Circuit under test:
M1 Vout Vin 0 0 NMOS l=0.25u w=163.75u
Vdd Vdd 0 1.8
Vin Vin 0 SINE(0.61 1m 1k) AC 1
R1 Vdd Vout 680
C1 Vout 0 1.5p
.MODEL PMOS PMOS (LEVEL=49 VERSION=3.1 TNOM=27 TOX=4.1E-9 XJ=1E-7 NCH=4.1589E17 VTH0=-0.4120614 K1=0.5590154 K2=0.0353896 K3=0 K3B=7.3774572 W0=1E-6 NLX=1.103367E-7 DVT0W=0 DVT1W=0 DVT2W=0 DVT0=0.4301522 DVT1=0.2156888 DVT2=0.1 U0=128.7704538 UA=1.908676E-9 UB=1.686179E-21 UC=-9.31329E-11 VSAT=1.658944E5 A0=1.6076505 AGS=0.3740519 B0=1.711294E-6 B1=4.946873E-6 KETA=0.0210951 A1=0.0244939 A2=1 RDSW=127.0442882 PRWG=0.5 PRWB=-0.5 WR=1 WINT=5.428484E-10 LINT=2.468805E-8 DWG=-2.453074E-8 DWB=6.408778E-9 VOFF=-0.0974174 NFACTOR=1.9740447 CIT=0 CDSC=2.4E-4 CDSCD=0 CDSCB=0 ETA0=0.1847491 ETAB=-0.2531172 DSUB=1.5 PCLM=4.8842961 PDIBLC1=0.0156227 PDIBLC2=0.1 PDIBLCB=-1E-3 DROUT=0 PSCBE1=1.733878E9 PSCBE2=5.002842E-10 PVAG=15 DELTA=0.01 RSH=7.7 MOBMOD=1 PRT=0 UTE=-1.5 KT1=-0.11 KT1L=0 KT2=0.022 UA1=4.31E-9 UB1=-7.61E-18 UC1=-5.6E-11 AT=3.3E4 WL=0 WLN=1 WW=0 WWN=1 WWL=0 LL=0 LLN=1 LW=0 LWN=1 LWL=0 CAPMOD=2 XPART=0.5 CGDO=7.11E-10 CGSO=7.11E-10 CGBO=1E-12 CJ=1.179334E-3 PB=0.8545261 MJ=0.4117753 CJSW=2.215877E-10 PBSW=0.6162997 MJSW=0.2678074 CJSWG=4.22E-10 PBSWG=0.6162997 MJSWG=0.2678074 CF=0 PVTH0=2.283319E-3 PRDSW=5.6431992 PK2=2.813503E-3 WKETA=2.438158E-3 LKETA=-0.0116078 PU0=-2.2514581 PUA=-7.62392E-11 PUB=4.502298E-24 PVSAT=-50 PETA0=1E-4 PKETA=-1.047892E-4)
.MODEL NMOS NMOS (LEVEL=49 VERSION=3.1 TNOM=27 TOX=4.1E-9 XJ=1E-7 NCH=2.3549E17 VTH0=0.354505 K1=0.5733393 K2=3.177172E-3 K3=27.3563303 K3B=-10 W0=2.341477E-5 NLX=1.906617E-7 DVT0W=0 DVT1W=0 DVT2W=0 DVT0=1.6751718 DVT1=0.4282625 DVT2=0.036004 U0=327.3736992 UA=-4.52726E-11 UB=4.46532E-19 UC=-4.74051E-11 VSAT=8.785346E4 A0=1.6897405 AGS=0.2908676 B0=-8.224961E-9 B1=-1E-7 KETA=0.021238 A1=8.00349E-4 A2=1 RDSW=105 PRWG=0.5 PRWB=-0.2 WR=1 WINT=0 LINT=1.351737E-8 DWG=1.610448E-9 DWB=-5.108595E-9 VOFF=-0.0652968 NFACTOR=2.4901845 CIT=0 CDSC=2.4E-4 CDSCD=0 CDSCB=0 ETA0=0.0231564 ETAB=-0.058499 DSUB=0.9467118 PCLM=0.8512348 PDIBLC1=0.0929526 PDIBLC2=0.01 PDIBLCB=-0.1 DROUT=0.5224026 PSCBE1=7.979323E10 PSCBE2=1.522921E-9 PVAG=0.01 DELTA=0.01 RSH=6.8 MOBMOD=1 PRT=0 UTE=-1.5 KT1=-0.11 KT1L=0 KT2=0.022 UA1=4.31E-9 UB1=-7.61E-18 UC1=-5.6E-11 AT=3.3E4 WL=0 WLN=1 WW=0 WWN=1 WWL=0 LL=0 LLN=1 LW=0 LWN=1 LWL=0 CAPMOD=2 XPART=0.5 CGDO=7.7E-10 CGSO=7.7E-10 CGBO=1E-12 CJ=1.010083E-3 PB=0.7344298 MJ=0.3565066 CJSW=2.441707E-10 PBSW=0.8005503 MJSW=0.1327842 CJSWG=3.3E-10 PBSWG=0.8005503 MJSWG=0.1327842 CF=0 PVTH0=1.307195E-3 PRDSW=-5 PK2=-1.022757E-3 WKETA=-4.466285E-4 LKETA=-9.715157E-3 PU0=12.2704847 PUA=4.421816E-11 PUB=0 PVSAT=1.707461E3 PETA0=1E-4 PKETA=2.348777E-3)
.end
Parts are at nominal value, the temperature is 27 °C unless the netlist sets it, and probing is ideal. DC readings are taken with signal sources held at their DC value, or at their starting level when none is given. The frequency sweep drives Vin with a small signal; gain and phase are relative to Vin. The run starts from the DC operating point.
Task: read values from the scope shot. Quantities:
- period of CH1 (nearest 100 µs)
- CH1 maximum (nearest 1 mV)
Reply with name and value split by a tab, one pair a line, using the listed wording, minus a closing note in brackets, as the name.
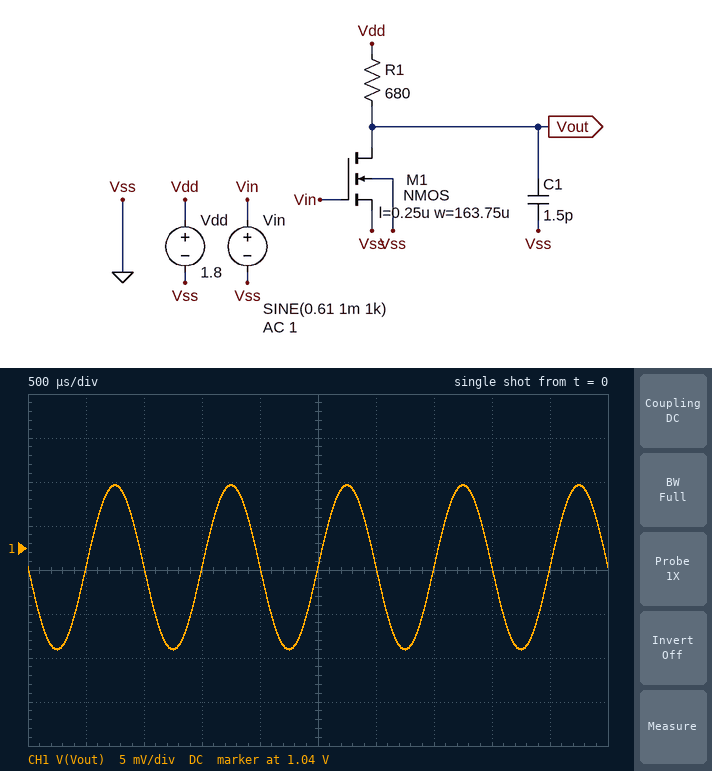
period of CH1	1.0 ms
CH1 maximum	1.047 V
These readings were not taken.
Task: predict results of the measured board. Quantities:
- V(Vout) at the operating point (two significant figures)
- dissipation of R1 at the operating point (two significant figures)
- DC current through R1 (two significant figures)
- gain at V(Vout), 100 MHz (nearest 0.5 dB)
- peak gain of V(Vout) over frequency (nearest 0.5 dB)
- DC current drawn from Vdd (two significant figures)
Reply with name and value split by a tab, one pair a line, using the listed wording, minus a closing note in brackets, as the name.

V(Vout) at the operating point	1.0 V
dissipation of R1 at the operating point	850 µW
DC current through R1	1.1 mA
gain at V(Vout), 100 MHz	18.0 dB
peak gain of V(Vout) over frequency	19.5 dB
DC current drawn from Vdd	1.1 mA
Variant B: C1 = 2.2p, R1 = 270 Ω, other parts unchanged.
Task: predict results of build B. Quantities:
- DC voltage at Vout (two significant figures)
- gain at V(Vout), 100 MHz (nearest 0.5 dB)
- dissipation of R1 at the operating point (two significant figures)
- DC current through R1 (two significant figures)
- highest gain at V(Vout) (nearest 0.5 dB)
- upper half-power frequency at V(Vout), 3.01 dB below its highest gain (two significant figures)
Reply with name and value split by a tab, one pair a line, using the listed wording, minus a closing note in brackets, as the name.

DC voltage at Vout	1.5 V
gain at V(Vout), 100 MHz	12.0 dB
dissipation of R1 at the operating point	390 µW
DC current through R1	1.2 mA
highest gain at V(Vout)	12.5 dB
upper half-power frequency at V(Vout), 3.01 dB below its highest gain	260 MHz
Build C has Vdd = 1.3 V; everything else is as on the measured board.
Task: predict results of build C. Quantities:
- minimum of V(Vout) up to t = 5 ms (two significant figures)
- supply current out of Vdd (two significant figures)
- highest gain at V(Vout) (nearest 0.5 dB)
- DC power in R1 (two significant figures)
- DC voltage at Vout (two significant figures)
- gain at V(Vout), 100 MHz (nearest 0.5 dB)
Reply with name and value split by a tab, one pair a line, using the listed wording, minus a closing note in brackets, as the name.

minimum of V(Vout) up to t = 5 ms	590 mV
supply current out of Vdd	1.0 mA
highest gain at V(Vout)	19.0 dB
DC power in R1	720 µW
DC voltage at Vout	600 mV
gain at V(Vout), 100 MHz	17.5 dB
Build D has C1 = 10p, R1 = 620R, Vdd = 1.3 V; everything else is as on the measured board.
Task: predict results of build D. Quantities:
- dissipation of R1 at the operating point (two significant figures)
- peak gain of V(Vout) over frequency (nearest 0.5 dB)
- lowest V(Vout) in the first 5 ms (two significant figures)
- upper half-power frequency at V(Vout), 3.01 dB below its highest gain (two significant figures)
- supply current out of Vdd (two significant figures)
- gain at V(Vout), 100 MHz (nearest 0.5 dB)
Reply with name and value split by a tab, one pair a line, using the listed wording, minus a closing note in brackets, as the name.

dissipation of R1 at the operating point	670 µW
peak gain of V(Vout) over frequency	18.0 dB
lowest V(Vout) in the first 5 ms	650 mV
upper half-power frequency at V(Vout), 3.01 dB below its highest gain	29 MHz
supply current out of Vdd	1.0 mA
gain at V(Vout), 100 MHz	7.0 dB
